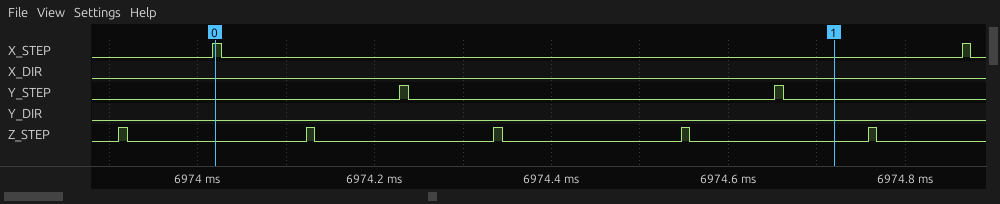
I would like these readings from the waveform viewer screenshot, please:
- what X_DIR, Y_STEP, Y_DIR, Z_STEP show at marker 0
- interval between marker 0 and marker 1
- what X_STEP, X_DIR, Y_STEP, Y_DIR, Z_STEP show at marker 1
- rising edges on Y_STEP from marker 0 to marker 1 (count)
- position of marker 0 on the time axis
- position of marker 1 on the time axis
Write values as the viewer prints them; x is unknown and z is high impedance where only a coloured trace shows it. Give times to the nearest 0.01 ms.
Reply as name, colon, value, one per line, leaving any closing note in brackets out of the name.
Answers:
what X_DIR, Y_STEP, Y_DIR, Z_STEP show at marker 0: X_DIR=0, Y_STEP=0, Y_DIR=0, Z_STEP=0
interval between marker 0 and marker 1: 0.7 ms
what X_STEP, X_DIR, Y_STEP, Y_DIR, Z_STEP show at marker 1: X_STEP=0, X_DIR=0, Y_STEP=0, Y_DIR=0, Z_STEP=0
rising edges on Y_STEP from marker 0 to marker 1: 2
position of marker 0 on the time axis: 6974.02 ms
position of marker 1 on the time axis: 6974.72 ms
